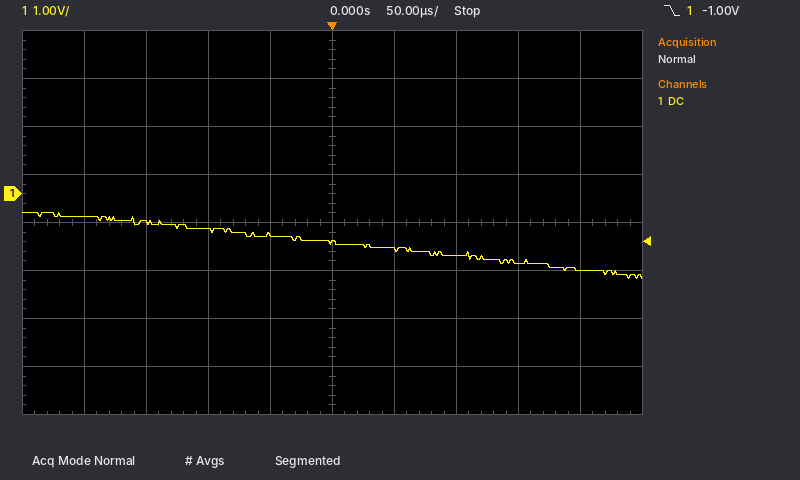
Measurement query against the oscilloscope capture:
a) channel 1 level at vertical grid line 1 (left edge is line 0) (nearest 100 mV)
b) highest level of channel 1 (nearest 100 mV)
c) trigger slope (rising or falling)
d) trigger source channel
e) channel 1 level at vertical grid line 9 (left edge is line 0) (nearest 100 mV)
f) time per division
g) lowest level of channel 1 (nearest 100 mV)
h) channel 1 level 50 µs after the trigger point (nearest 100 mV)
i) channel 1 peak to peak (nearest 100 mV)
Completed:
-500 mV
-400 mV
falling
channel 1
-1.6 V
50 µs
-1.8 V
-1.2 V
1.4 V
